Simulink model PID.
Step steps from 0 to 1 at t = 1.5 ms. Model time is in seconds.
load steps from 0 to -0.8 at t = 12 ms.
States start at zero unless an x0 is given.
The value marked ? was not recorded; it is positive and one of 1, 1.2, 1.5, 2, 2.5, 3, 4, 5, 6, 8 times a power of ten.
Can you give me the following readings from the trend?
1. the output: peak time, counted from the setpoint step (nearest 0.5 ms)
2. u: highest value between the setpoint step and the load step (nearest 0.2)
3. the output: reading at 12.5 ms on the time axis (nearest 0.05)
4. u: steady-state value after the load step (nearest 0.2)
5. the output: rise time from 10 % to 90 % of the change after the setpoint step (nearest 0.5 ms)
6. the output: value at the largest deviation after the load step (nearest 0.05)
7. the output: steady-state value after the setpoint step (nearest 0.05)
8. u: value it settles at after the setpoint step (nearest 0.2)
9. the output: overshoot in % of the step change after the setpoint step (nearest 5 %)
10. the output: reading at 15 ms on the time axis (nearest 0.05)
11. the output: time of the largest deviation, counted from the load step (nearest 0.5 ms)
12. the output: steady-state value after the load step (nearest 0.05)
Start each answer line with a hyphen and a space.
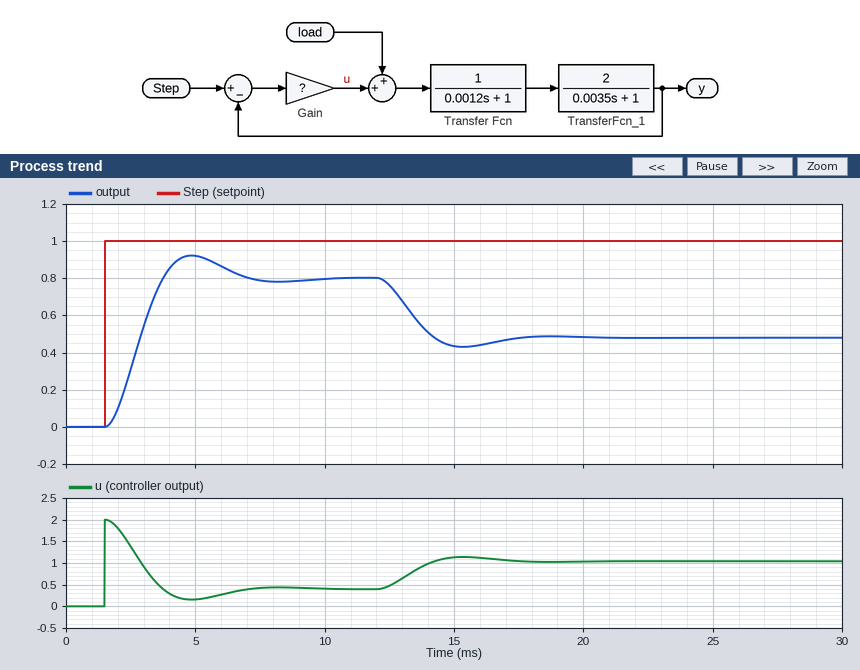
- 3.5 ms
- 2.0
- 0.75
- 1.0
- 1.5 ms
- 0.45
- 0.80
- 0.4
- 15 %
- 0.45
- 3.5 ms
- 0.50
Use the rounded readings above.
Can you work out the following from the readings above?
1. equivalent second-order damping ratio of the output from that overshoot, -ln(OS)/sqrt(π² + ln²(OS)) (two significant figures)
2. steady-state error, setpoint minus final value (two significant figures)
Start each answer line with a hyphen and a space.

- 0.52
- 0.20
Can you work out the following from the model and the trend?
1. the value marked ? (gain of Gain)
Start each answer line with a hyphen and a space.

- 2
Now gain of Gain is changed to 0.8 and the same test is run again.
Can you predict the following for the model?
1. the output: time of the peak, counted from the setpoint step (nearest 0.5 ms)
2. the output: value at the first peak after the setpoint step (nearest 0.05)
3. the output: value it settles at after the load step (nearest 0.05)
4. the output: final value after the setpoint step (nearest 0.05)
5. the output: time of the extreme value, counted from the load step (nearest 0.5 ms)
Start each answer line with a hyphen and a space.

- 5.5 ms
- 0.65
- 0.00
- 0.60
- 5.5 ms
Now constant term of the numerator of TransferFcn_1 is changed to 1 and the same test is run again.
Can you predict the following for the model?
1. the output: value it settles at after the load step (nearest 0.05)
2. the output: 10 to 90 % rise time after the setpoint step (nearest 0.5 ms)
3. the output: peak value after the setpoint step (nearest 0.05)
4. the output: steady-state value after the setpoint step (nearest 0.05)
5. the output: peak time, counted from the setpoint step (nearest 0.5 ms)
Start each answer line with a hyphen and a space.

- 0.40
- 2.5 ms
- 0.70
- 0.65
- 5.0 ms
